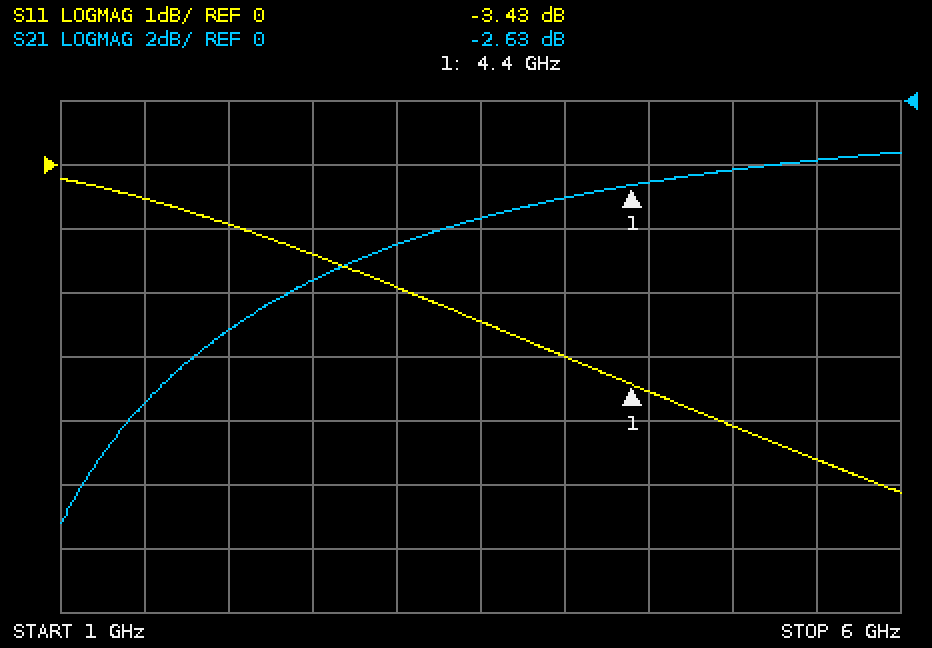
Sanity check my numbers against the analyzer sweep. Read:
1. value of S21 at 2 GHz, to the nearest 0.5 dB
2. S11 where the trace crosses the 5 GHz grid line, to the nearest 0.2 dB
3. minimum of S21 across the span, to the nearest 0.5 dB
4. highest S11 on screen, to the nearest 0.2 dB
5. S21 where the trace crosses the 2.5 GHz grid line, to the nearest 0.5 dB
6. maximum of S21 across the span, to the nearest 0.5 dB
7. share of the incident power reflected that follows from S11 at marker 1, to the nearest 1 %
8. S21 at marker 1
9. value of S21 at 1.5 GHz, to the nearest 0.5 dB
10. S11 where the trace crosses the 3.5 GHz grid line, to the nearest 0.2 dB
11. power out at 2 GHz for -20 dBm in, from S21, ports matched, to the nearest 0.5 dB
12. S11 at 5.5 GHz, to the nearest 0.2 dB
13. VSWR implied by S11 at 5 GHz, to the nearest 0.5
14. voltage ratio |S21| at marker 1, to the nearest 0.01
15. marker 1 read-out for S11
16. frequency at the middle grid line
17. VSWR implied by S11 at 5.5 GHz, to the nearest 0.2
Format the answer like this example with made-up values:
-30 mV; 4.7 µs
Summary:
-7.0 dB; -4.0 dB; -13.0 dB; -0.2 dB; -5.5 dB; -1.5 dB; 45 %; -2.63 dB; -9.5 dB; -2.4 dB; -27.0 dBm; -4.6 dB; 4.5; 0.74; -3.43 dB; 3.5 GHz; 3.8
